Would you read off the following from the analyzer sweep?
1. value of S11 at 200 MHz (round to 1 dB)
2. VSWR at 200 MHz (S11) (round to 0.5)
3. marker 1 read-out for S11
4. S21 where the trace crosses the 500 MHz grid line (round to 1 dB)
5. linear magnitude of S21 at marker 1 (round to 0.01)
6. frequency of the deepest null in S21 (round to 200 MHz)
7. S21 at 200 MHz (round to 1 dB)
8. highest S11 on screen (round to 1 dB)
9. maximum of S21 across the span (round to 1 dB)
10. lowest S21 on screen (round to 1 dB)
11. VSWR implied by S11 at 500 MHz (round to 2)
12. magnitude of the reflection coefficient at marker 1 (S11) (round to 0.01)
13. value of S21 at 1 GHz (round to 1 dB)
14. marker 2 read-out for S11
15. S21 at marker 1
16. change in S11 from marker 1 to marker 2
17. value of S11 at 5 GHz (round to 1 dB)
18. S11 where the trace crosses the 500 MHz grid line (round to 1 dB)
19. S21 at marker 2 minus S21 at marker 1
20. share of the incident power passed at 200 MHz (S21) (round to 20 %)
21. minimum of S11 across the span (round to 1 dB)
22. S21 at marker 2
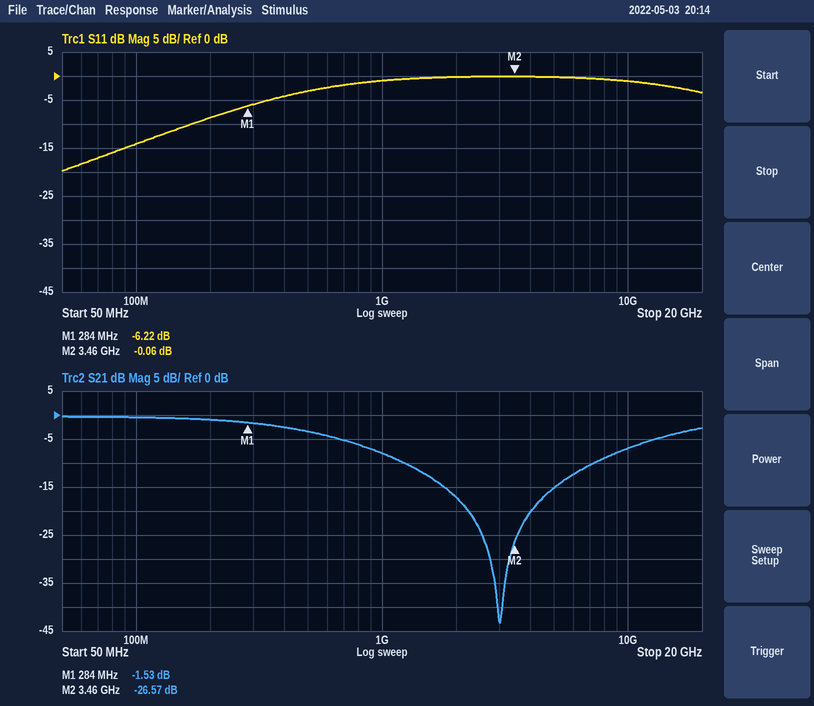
-9 dB
2.0
-6.22 dB
-3 dB
0.84
3.0 GHz
-1 dB
0 dB
0 dB
-43 dB
6
0.49
-8 dB
-0.06 dB
-1.53 dB
6.16 dB
0 dB
-3 dB
-25.04 dB
80 %
-20 dB
-26.57 dB
